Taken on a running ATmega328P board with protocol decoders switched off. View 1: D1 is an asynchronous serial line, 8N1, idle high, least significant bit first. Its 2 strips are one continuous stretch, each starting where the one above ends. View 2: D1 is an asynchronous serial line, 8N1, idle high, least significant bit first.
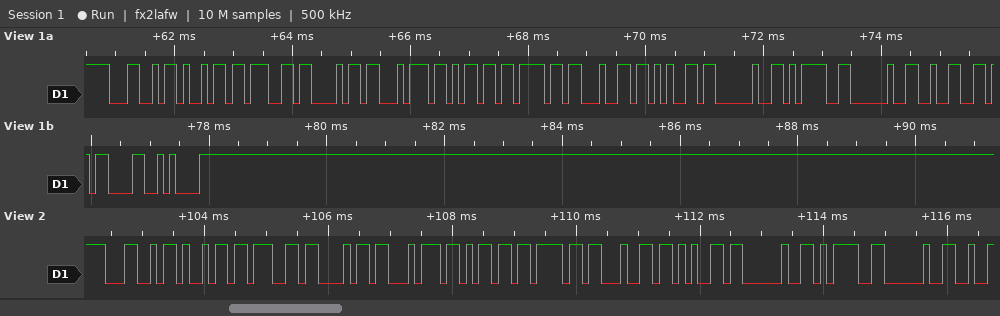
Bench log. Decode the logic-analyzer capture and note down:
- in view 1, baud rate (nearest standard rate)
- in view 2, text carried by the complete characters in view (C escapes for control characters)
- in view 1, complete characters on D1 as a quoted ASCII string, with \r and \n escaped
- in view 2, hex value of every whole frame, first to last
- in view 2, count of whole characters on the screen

9600 baud
"Lightmode = "
"Lightmode = 2\r\n"
4C 69 67 68 74 6D 6F 64 65 20 3D 20
12
